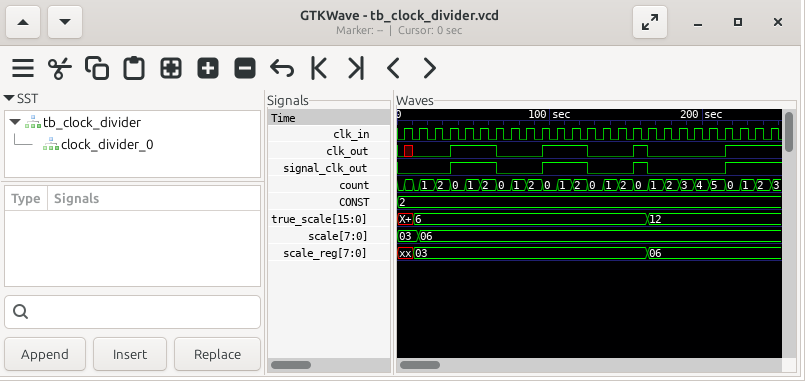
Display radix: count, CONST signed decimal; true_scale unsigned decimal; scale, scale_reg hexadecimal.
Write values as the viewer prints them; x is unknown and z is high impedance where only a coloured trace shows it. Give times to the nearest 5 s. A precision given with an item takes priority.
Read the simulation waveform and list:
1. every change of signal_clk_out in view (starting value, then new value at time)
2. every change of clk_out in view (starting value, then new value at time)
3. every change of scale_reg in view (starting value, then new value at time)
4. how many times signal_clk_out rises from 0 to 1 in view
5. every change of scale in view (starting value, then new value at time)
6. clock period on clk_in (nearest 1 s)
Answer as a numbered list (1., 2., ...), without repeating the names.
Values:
1. 0, 1 at 35 s, 0 at 65 s, 1 at 95 s, 0 at 125 s, 1 at 155 s, 0 at 165 s, 1 at 215 s
2. 0, x at 5 s, 0 at 10 s, 1 at 35 s, 0 at 65 s, 1 at 95 s, 0 at 125 s, 1 at 155 s, 0 at 165 s, 1 at 215 s
3. xx, 03 at 10 s, 06 at 165 s
4. 4
5. 03, 06 at 15 s
6. 10 s
